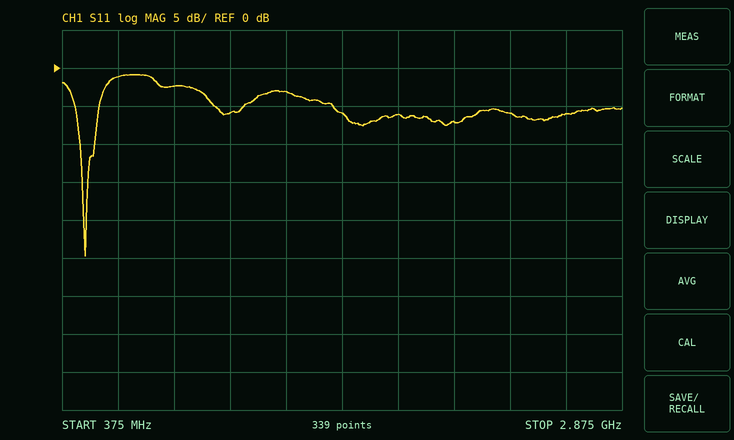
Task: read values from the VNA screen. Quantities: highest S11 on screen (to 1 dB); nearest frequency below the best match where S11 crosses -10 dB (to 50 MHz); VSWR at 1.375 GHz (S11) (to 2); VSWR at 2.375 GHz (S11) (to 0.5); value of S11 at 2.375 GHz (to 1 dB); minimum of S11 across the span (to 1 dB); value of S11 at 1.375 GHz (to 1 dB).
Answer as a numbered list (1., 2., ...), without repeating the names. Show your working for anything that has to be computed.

1. -1 dB
2. 450 MHz
3. |Γ| = 10^(-3/20) = 0.7079; VSWR = (1 + 0.7079)/(1 − 0.7079) ≈ 6
4. |Γ| = 10^(-6/20) = 0.5012; VSWR = (1 + 0.5012)/(1 − 0.5012) ≈ 3.0
5. -6 dB
6. -25 dB
7. -3 dB
